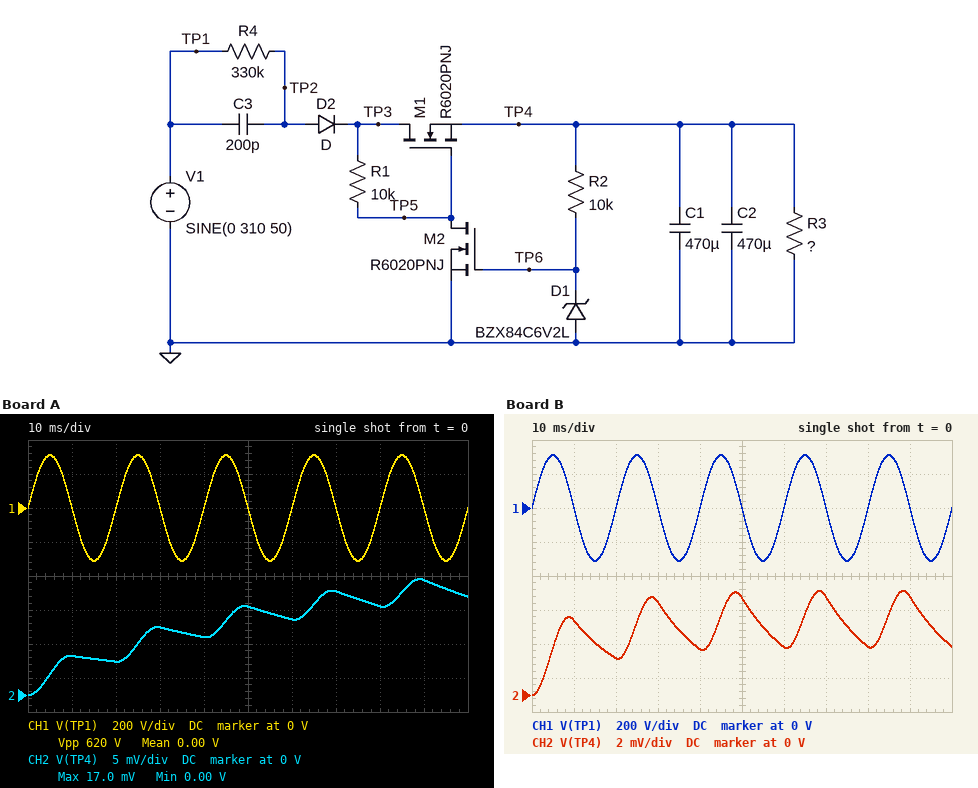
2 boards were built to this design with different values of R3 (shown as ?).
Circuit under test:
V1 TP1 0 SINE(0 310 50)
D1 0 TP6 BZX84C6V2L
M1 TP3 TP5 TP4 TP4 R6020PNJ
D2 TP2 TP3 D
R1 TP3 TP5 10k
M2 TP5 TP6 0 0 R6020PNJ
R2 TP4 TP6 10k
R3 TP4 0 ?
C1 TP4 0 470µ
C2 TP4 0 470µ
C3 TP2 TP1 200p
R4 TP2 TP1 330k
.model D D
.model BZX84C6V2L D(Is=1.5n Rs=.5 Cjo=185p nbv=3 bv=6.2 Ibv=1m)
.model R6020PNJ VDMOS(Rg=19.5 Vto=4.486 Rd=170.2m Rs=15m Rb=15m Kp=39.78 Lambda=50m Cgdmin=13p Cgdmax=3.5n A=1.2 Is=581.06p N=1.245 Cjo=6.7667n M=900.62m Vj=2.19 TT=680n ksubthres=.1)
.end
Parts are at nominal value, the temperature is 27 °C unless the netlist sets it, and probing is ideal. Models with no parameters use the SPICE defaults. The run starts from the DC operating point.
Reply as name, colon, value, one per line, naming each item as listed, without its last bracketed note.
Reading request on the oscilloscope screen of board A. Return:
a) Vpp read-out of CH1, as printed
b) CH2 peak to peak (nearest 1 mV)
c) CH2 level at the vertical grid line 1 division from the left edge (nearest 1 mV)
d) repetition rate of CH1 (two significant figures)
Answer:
Vpp read-out of CH1, as printed: 620 V
CH2 peak to peak: 17 mV
CH2 level at the vertical grid line 1 division from the left edge: 6 mV
repetition rate of CH1: 50 Hz
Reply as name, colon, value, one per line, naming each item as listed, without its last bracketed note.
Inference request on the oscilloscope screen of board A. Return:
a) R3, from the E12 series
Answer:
R3, from the E12 series: 68 Ω
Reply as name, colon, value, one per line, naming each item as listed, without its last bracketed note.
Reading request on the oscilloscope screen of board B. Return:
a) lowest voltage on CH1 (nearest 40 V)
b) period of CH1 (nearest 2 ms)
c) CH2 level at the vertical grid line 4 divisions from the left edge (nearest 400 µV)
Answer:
lowest voltage on CH1: -320 V
period of CH1: 20 ms
CH2 level at the vertical grid line 4 divisions from the left edge: 2.8 mV
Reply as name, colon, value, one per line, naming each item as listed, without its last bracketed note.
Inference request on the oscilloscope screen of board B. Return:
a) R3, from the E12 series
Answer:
R3, from the E12 series: 15 Ω
